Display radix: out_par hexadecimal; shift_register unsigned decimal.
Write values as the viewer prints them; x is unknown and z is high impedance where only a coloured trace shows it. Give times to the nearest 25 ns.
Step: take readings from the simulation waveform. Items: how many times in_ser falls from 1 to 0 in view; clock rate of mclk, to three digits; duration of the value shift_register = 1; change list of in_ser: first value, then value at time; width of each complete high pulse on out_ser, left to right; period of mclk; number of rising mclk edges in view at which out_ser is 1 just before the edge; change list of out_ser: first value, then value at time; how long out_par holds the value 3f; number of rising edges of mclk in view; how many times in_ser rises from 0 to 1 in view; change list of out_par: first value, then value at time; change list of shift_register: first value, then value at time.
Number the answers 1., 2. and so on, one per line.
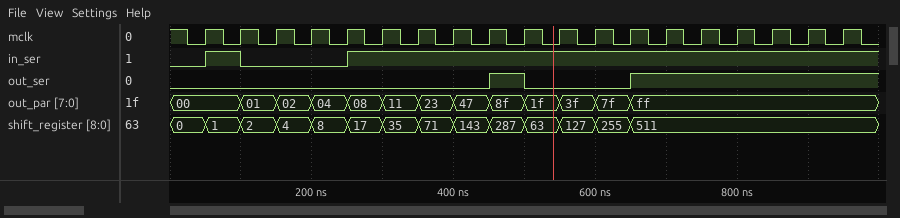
1. 1
2. 20.0 MHz
3. 50 ns
4. 0, 1 at 50 ns, 0 at 100 ns, 1 at 250 ns
5. 50 ns
6. 50 ns
7. 7
8. 0, 1 at 450 ns, 0 at 500 ns, 1 at 650 ns
9. 50 ns
10. 19
11. 2
12. 00, 01 at 100 ns, 02 at 150 ns, 04 at 200 ns, 08 at 250 ns, 11 at 300 ns, 23 at 350 ns, 47 at 400 ns, 8f at 450 ns, 1f at 500 ns, 3f at 550 ns, 7f at 600 ns, ff at 650 ns
13. 0, 1 at 50 ns, 2 at 100 ns, 4 at 150 ns, 8 at 200 ns, 17 at 250 ns, 35 at 300 ns, 71 at 350 ns, 143 at 400 ns, 287 at 450 ns, 63 at 500 ns, 127 at 550 ns, 255 at 600 ns, 511 at 650 ns
